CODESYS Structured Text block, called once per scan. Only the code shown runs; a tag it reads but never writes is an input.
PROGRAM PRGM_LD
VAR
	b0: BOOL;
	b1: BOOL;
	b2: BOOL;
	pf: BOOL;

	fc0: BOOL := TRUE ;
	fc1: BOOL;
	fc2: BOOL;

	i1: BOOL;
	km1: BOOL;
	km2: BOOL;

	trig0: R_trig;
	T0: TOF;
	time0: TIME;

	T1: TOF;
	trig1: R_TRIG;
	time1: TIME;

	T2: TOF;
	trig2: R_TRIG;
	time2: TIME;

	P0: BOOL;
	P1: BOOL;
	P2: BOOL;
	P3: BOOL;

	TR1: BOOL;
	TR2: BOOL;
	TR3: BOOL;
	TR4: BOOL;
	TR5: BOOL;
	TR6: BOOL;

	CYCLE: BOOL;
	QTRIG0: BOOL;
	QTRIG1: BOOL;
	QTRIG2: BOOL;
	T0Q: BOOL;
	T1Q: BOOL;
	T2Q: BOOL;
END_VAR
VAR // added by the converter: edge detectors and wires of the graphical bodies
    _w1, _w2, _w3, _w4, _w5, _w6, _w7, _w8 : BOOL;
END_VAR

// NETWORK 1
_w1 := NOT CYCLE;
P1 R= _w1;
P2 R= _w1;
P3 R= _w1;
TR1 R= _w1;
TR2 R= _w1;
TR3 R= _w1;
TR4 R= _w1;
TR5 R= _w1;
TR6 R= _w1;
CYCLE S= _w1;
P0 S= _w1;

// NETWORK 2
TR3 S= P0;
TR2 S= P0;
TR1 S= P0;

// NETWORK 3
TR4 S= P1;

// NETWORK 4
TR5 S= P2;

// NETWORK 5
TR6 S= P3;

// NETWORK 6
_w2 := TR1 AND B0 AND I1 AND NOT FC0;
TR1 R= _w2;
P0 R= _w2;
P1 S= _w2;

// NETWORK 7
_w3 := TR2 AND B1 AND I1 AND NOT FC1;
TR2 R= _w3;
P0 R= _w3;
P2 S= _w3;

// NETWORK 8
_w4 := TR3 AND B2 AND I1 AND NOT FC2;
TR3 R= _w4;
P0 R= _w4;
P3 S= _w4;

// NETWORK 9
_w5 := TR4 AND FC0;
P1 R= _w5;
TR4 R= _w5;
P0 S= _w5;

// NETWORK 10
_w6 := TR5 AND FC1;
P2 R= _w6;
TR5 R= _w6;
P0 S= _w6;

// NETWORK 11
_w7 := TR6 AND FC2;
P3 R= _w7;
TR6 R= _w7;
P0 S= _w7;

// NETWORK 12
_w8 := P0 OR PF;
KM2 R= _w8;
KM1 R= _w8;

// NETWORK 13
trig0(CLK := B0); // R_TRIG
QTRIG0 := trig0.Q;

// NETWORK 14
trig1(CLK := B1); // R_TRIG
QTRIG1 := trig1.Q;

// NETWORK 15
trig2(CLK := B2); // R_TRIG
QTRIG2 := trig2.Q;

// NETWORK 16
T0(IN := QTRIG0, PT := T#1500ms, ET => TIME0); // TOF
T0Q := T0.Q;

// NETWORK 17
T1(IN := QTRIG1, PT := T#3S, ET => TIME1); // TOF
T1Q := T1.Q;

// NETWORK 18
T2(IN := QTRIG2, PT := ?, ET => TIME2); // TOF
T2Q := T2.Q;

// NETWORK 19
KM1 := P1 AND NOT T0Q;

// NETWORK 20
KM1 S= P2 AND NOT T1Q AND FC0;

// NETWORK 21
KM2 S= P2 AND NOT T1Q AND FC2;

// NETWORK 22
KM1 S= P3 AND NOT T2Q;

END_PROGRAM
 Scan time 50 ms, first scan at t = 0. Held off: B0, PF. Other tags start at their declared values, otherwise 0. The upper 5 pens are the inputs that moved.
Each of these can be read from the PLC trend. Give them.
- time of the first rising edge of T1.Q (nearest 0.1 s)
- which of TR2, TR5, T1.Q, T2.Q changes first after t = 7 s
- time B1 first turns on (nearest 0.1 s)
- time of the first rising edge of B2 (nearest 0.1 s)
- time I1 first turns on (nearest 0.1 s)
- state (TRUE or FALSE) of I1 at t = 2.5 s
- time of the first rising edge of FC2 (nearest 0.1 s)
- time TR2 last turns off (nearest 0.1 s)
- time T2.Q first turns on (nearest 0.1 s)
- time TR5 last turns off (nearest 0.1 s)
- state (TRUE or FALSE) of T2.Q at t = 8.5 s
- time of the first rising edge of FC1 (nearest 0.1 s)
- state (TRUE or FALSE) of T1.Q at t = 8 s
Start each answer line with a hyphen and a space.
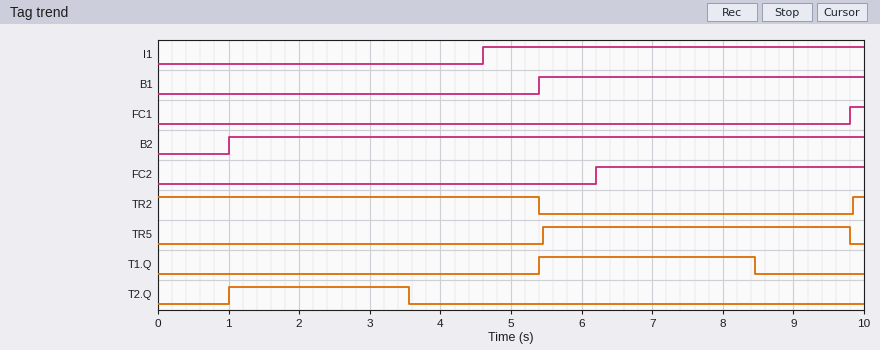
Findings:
- 5.4 s
- T1.Q
- 5.4 s
- 1.0 s
- 4.6 s
- FALSE
- 6.2 s
- 5.4 s
- 1.0 s
- 9.8 s
- FALSE
- 9.8 s
- TRUE
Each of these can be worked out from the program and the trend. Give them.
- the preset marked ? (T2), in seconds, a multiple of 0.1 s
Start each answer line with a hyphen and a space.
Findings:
- 2.5 s
